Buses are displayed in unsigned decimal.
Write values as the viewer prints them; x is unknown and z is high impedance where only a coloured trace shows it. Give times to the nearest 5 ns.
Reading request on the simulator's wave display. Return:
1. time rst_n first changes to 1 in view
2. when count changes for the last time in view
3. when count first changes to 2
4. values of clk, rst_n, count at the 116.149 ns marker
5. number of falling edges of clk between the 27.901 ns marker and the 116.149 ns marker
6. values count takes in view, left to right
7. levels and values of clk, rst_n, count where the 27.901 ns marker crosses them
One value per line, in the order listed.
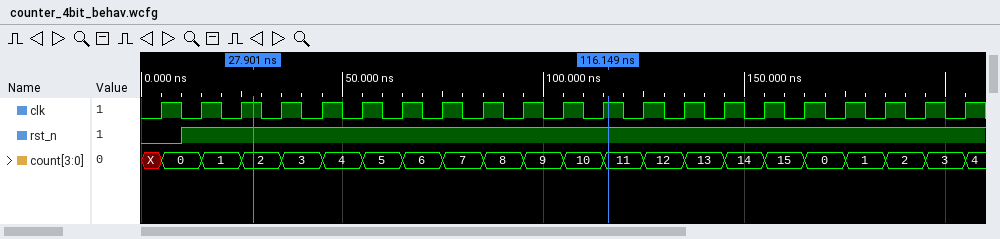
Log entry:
10 ns
205 ns
25 ns
clk=1, rst_n=1, count=11
9
X, 0, 1, 2, 3, 4, 5, 6, 7, 8, 9, 10, 11, 12, 13, 14, 15, 0, 1, 2, 3, 4
clk=1, rst_n=1, count=2
